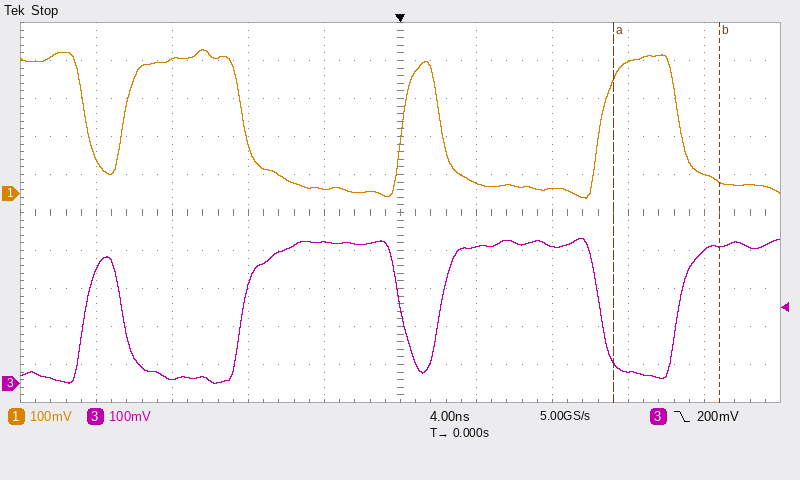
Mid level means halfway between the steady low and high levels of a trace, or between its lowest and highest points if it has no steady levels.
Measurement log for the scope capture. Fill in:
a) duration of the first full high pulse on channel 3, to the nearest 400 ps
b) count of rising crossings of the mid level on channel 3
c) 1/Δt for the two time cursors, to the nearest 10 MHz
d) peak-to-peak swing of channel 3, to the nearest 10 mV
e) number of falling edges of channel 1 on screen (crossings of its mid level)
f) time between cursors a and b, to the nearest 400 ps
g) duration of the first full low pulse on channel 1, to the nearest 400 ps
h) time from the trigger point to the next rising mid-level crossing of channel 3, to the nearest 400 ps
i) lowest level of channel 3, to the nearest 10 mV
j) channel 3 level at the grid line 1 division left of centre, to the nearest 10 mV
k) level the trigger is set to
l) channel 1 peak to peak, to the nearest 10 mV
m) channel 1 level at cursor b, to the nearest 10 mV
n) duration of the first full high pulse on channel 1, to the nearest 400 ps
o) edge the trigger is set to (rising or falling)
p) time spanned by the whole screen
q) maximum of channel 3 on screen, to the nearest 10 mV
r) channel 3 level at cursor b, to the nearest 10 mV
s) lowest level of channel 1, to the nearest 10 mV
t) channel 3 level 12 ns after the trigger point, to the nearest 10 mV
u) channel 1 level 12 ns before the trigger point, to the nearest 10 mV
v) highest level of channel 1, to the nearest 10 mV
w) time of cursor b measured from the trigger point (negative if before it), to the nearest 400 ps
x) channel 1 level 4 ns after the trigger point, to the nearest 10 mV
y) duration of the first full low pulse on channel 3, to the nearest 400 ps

2.0 ns
4
180 MHz
380 mV
4
5.6 ns
2.0 ns
2.0 ns
0 mV
370 mV
200 mV
390 mV
30 mV
6.4 ns
falling
40 ns
380 mV
360 mV
-10 mV
30 mV
350 mV
380 mV
+16.8 ns
30 mV
6.4 ns
